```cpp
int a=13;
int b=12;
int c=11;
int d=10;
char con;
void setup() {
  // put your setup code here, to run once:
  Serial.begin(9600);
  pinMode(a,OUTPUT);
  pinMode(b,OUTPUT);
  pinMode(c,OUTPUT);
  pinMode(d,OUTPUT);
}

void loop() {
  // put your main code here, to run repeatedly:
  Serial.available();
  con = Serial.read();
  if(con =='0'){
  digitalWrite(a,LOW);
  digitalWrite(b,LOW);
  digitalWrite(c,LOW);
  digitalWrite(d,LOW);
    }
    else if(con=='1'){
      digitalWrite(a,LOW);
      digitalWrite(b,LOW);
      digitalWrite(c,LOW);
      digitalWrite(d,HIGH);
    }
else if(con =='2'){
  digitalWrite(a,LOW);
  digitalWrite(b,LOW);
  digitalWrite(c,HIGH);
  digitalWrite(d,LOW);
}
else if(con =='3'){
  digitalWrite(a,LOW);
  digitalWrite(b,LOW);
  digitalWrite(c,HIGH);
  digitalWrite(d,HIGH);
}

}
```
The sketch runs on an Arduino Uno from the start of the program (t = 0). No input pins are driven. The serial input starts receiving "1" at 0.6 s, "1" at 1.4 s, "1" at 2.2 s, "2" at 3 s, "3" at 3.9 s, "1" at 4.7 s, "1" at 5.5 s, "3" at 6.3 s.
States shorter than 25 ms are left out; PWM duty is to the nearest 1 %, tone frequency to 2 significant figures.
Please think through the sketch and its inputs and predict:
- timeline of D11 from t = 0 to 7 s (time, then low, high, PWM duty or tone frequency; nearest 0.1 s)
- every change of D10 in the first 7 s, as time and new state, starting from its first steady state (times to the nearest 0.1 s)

0 s low; 3 s high; 4.7 s low; 6.3 s high
0 s low; 0.6 s high; 3 s low; 3.9 s high
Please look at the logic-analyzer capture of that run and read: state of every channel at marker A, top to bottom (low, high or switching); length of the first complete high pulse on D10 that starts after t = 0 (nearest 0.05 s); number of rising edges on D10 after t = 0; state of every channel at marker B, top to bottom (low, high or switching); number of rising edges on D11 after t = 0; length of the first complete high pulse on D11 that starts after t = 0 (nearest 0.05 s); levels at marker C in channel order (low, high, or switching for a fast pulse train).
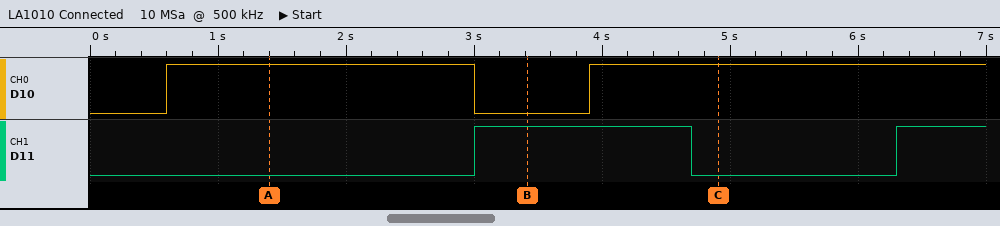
D10 high, D11 low
2.40 s
2
D10 low, D11 high
2
1.70 s
D10 high, D11 low
